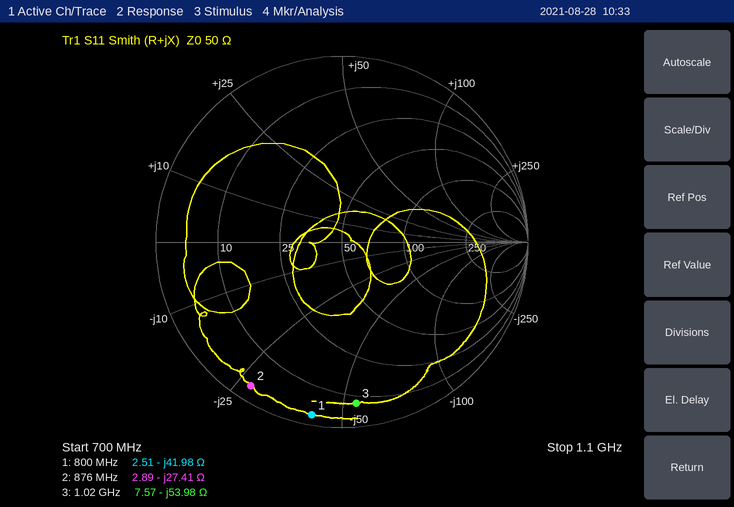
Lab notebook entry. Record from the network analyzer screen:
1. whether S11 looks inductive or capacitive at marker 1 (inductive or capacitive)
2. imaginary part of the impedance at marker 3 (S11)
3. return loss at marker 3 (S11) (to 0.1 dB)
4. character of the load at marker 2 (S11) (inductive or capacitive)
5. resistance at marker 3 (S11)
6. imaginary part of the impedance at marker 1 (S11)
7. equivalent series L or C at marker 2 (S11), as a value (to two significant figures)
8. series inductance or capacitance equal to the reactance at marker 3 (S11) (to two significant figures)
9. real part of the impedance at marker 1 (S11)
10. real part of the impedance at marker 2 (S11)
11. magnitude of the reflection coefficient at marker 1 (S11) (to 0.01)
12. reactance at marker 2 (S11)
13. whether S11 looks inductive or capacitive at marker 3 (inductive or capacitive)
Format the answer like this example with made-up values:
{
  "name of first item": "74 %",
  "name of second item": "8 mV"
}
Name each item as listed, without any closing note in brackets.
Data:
{
  "whether S11 looks inductive or capacitive at marker 1": "capacitive",
  "imaginary part of the impedance at marker 3": "-53.98 Ω",
  "return loss at marker 3 (S11)": "1.2 dB",
  "character of the load at marker 2 (S11)": "capacitive",
  "resistance at marker 3": "7.57 Ω",
  "imaginary part of the impedance at marker 1": "-41.98 Ω",
  "equivalent series L or C at marker 2 (S11), as a value": "6.6 pF",
  "series inductance or capacitance equal to the reactance at marker 3 (S11)": "2.9 pF",
  "real part of the impedance at marker 1": "2.51 Ω",
  "real part of the impedance at marker 2": "2.89 Ω",
  "magnitude of the reflection coefficient at marker 1 (S11)": "0.94",
  "reactance at marker 2": "-27.41 Ω",
  "whether S11 looks inductive or capacitive at marker 3": "capacitive"
}
